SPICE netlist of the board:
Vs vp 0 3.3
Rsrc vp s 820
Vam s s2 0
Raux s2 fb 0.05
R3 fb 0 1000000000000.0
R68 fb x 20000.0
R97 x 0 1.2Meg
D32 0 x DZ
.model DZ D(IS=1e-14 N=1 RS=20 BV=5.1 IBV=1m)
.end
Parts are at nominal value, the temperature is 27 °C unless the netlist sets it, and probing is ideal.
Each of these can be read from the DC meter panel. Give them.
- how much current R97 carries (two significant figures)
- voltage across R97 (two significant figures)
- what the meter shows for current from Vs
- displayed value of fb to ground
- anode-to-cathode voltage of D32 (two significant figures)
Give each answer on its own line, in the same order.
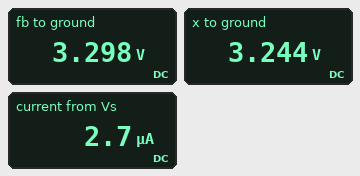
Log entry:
2.7 µA
3.2 V
2.7 µA
3.298 V
-3.2 V
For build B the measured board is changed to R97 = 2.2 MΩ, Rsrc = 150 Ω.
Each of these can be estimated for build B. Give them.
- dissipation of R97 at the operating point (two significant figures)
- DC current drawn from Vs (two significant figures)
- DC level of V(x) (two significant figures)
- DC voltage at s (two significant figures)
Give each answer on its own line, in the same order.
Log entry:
4.9 µW
1.5 µA
3.3 V
3.3 V
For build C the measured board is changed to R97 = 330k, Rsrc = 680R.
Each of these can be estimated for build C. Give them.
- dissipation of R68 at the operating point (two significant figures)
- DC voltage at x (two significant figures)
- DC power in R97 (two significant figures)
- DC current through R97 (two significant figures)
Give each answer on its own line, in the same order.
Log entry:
1.8 µW
3.1 V
29 µW
9.4 µA
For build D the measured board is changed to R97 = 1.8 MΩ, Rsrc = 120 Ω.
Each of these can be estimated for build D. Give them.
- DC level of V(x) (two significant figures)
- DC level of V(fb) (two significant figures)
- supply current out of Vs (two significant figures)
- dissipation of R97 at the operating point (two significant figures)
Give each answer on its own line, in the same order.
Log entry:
3.3 V
3.3 V
1.8 µA
5.9 µW
